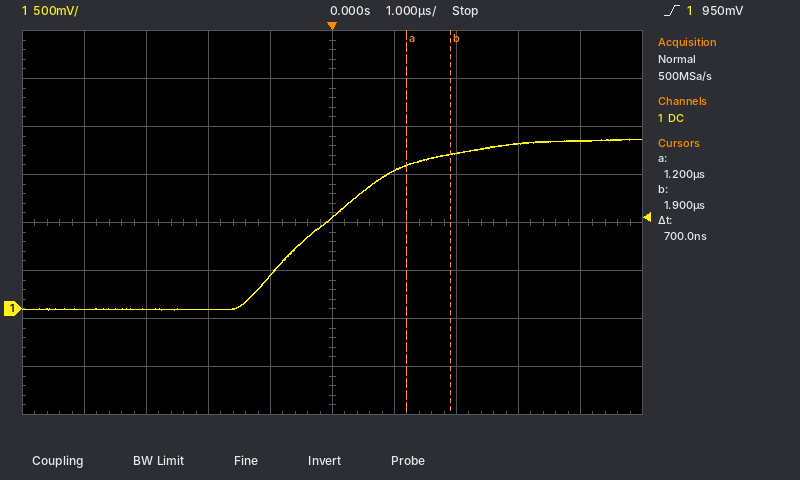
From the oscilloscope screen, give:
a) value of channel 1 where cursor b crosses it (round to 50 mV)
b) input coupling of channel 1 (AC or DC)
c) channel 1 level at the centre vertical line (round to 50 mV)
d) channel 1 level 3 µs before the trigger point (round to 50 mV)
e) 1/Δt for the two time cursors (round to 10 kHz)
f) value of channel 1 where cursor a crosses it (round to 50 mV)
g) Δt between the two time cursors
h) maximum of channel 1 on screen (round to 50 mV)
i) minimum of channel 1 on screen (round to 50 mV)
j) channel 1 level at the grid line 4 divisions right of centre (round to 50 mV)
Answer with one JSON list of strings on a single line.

["1.60 V", "DC", "950 mV", "0 mV", "1.43 MHz", "1.50 V", "700 ns", "1.75 V", "0 mV", "1.75 V"]
